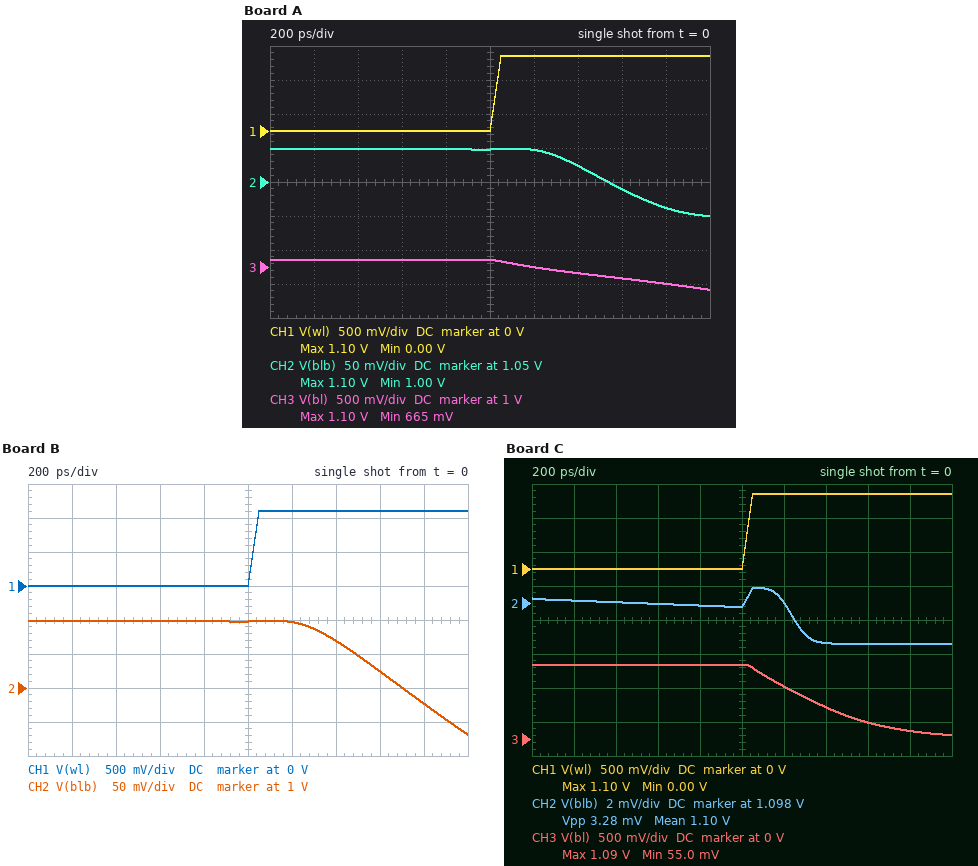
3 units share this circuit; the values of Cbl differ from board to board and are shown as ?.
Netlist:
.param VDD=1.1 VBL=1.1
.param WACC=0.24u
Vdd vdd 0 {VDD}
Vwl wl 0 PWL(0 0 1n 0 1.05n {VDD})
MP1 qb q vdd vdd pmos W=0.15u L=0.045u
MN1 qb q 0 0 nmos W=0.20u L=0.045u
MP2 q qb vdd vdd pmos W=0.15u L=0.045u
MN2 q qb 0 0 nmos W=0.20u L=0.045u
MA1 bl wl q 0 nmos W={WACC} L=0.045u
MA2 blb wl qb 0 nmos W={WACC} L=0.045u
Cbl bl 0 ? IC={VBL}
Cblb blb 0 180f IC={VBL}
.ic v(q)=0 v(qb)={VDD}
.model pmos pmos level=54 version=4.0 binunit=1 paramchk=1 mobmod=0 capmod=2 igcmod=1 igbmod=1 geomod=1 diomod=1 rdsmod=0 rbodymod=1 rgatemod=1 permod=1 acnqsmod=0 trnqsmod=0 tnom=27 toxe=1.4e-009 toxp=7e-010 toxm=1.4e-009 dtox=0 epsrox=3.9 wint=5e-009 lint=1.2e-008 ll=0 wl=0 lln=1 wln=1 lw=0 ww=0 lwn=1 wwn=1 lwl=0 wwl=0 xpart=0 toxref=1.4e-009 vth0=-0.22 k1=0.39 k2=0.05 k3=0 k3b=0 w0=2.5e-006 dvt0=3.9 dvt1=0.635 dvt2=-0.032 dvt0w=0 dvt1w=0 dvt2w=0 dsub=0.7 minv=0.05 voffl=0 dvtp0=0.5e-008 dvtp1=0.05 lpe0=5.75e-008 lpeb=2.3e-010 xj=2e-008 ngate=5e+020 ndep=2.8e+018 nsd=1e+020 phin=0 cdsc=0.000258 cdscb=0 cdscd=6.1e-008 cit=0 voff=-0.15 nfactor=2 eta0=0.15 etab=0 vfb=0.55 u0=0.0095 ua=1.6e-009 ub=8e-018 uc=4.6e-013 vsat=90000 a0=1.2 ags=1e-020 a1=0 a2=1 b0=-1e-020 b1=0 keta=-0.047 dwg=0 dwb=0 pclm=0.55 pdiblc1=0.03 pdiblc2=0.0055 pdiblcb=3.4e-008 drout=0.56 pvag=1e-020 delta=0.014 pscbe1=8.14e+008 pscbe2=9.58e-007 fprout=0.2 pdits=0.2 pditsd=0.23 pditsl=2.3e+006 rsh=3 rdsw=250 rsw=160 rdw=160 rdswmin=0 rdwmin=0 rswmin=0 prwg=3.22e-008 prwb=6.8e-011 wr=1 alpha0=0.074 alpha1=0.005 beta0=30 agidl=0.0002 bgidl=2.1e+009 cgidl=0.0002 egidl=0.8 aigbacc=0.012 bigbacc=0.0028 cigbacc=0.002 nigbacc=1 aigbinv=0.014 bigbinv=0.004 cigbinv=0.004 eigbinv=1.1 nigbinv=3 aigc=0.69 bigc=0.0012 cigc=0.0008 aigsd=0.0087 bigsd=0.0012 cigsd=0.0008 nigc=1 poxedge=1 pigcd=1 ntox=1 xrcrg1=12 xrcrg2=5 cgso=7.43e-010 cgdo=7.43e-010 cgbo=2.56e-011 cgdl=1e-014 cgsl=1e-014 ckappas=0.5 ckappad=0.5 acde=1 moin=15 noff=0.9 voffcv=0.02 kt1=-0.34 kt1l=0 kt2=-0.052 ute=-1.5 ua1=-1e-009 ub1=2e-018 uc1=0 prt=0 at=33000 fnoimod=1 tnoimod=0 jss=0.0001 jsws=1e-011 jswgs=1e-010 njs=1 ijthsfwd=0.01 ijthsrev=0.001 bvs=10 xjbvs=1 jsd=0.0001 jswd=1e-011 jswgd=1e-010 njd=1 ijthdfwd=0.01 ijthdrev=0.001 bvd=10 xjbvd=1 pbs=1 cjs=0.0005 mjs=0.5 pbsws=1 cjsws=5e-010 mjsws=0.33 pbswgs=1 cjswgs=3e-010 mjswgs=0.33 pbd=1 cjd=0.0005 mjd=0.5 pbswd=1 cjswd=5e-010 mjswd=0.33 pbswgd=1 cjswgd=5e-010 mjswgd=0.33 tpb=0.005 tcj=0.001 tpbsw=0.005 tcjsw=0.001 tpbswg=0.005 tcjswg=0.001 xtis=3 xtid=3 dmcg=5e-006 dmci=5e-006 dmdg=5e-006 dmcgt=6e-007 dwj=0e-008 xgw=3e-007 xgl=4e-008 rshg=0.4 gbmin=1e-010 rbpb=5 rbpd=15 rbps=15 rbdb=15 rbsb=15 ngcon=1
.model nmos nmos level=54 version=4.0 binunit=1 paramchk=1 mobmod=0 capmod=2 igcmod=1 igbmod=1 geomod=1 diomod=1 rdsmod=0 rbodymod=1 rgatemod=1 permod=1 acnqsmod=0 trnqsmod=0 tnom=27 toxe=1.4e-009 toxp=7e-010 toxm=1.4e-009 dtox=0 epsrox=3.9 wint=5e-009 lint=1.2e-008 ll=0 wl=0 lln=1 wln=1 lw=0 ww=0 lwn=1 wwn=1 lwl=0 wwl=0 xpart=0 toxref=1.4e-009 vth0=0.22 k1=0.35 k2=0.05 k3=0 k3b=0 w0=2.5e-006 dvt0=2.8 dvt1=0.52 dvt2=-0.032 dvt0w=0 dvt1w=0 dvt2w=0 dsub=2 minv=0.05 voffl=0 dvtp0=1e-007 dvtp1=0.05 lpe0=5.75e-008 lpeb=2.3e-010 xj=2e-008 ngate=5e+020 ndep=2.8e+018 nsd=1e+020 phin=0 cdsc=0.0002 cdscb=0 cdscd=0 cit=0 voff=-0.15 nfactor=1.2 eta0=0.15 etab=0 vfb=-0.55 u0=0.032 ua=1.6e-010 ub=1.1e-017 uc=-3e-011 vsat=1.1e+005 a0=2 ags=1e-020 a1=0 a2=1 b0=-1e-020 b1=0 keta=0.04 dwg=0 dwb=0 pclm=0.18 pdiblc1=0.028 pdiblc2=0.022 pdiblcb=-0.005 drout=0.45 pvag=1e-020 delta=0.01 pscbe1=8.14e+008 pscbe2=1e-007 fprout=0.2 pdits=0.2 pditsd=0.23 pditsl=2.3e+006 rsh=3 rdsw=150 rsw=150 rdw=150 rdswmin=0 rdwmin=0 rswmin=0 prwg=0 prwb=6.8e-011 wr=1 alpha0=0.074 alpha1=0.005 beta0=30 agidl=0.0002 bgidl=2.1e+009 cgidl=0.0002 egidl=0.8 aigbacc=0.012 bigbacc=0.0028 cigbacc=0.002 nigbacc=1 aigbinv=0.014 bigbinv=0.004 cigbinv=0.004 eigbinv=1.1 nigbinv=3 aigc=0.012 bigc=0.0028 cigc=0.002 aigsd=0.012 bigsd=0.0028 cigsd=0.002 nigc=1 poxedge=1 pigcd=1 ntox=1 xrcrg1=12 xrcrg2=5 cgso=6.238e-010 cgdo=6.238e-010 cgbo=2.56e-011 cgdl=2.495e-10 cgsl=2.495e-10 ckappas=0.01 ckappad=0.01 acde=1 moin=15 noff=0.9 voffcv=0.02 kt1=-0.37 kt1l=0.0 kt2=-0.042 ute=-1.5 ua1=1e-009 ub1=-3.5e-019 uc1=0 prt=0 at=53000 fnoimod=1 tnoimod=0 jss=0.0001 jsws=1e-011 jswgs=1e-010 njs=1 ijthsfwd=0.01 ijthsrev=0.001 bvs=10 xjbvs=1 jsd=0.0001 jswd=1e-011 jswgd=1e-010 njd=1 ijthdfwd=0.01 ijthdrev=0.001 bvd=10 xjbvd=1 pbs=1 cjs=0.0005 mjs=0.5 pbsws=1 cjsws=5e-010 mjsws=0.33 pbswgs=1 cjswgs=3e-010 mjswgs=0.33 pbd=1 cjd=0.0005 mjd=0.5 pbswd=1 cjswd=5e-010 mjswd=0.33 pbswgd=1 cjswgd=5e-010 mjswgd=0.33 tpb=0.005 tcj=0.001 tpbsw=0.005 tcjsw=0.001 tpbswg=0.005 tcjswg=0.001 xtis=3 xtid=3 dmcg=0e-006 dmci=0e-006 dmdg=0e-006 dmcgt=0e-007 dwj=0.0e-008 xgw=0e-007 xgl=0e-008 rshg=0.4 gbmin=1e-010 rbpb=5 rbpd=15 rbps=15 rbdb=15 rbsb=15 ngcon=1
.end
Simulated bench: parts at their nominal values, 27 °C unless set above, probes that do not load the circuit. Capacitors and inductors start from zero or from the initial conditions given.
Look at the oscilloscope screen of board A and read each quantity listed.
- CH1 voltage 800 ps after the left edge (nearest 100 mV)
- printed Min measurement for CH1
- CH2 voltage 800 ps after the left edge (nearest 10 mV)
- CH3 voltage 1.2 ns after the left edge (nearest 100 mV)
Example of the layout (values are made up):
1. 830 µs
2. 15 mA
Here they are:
1. 0 V
2. 0.00 V
3. 1.10 V
4. 1.0 V
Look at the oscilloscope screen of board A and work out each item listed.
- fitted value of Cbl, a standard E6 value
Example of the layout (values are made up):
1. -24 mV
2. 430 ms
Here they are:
1. 220 fF
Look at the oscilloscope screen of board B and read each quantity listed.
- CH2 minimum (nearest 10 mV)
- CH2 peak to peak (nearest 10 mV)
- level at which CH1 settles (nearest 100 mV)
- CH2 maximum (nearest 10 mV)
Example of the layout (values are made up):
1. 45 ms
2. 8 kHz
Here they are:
1. 930 mV
2. 170 mV
3. 1.1 V
4. 1.10 V
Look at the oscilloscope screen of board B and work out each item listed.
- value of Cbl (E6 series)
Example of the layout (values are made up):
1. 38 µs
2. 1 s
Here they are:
1. 330 fF
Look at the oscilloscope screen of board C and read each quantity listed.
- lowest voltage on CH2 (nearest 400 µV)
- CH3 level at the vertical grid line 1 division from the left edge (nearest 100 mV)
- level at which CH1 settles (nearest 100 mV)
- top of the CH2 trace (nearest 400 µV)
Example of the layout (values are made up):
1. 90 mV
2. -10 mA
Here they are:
1. 1.0956 V
2. 1.1 V
3. 1.1 V
4. 1.0988 V
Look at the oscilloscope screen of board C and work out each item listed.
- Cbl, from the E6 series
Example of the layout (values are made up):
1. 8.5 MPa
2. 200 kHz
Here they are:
1. 68 fF
